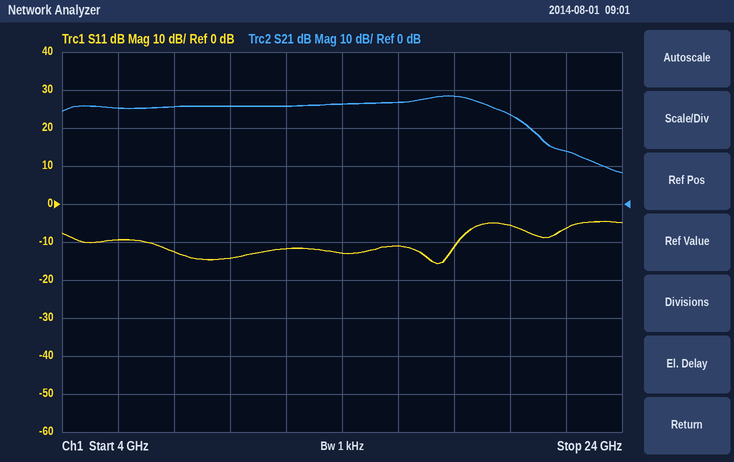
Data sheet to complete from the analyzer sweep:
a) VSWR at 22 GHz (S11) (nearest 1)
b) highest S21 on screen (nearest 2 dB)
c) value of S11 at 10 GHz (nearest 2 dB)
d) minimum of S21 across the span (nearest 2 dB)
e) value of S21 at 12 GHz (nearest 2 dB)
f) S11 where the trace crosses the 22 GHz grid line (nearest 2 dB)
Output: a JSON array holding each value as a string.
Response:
["3", "28 dB", "-14 dB", "8 dB", "26 dB", "-6 dB"]
